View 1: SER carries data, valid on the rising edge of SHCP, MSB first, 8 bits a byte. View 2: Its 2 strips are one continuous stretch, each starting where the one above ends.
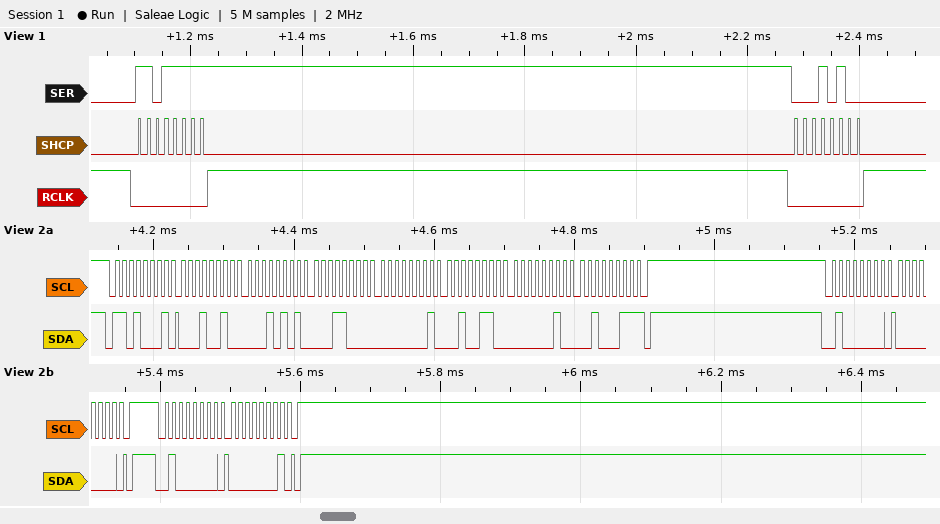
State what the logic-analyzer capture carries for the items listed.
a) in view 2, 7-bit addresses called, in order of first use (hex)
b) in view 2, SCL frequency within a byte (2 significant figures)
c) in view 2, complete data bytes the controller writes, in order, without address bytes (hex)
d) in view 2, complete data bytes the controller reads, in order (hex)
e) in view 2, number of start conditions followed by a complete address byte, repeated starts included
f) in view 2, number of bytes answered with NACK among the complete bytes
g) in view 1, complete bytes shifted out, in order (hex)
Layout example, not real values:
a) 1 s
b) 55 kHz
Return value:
a) 0x68 0x20
b) 100 kHz
c) 00 01
d) 12 15 18 01 26 02 23
e) 3
f) 1
g) 0xDF 0x14
